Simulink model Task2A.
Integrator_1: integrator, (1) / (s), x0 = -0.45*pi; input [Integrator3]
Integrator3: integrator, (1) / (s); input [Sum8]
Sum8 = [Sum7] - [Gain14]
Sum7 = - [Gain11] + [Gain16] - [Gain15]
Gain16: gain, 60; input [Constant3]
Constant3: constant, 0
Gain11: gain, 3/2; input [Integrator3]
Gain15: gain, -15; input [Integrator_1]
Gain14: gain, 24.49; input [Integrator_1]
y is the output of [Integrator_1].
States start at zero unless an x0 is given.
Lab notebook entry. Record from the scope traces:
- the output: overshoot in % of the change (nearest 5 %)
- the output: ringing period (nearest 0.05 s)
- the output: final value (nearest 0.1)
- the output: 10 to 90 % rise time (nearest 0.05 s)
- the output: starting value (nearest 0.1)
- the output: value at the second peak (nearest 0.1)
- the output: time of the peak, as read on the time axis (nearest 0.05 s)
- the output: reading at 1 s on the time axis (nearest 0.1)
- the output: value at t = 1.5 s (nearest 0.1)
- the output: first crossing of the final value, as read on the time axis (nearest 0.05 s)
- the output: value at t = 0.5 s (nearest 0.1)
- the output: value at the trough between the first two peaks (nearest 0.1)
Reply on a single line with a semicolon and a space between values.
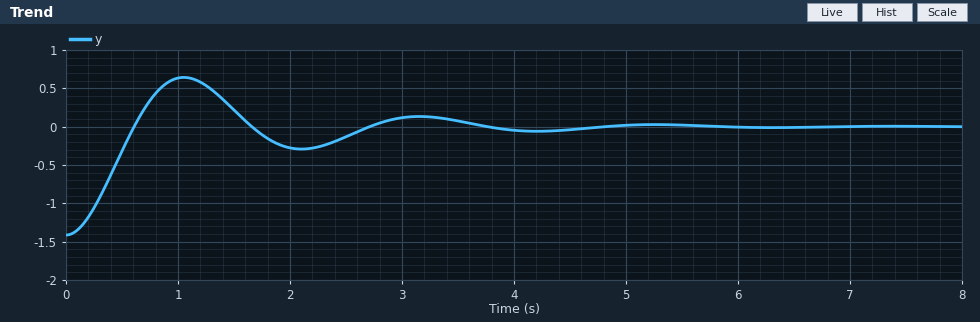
45 %; 2.10 s; 0.0; 0.40 s; -1.4; 0.1; 1.05 s; 0.6; 0.2; 0.60 s; -0.3; -0.3
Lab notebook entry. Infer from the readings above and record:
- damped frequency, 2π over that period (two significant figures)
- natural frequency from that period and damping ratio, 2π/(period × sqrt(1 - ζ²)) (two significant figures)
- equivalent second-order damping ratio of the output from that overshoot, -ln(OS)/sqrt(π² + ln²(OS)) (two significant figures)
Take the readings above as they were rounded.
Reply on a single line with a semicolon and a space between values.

3.0 rad/s; 3.1 rad/s; 0.25
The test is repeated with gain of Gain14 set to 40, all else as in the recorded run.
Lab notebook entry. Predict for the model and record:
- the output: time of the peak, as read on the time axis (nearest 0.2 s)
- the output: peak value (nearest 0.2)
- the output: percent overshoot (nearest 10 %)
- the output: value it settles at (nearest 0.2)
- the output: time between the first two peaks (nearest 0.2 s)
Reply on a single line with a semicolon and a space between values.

0.6 s; 0.8; 60 %; 0.0; 1.2 s
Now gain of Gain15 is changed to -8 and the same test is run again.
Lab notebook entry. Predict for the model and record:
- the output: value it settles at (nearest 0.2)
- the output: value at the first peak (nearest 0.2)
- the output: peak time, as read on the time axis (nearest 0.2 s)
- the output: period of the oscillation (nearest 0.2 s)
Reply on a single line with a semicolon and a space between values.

0.0; 0.8; 0.8 s; 1.6 s
